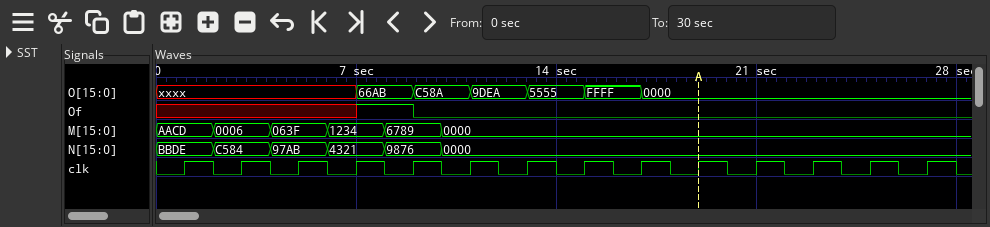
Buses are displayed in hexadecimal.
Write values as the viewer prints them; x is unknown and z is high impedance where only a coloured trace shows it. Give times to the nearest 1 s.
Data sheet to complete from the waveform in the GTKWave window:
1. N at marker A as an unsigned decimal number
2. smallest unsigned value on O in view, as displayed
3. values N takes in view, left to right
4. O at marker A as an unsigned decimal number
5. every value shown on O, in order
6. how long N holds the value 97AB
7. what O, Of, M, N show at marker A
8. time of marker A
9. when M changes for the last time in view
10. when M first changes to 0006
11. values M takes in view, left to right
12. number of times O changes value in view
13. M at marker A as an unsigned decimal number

0
0000
BBDE, C584, 97AB, 4321, 9876, 0000
0
xxxx, 66AB, C58A, 9DEA, 5555, FFFF, 0000
2 s
O=0000, Of=0, M=0000, N=0000
19 s
10 s
2 s
AACD, 0006, 063F, 1234, 6789, 0000
6
0
